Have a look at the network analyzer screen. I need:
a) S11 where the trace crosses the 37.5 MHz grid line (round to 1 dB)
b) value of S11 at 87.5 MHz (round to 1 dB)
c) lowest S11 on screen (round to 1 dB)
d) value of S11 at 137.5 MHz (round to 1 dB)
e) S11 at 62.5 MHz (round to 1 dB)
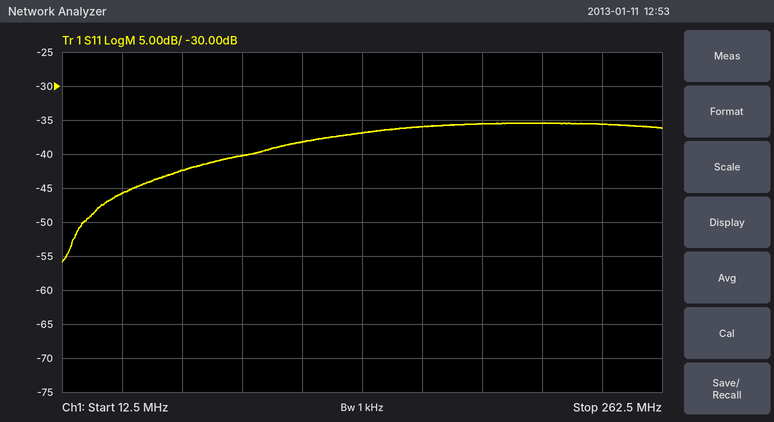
-46 dB
-40 dB
-56 dB
-37 dB
-42 dB
